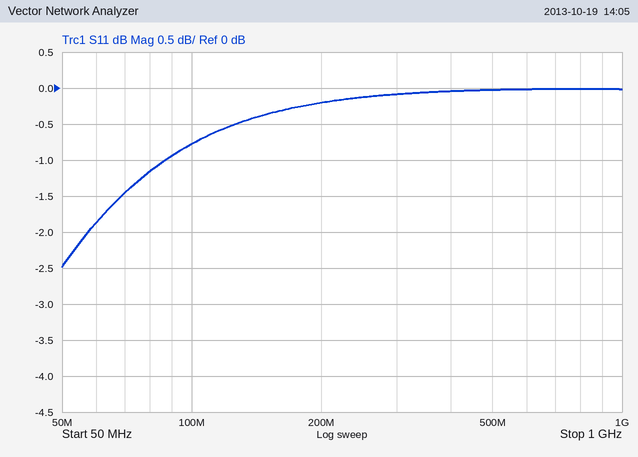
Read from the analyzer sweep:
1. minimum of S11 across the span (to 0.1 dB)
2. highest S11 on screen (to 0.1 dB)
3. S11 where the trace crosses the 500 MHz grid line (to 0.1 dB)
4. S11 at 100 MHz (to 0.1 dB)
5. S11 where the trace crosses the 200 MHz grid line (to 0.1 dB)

-2.5 dB
0.0 dB
0.0 dB
-0.8 dB
-0.2 dB
